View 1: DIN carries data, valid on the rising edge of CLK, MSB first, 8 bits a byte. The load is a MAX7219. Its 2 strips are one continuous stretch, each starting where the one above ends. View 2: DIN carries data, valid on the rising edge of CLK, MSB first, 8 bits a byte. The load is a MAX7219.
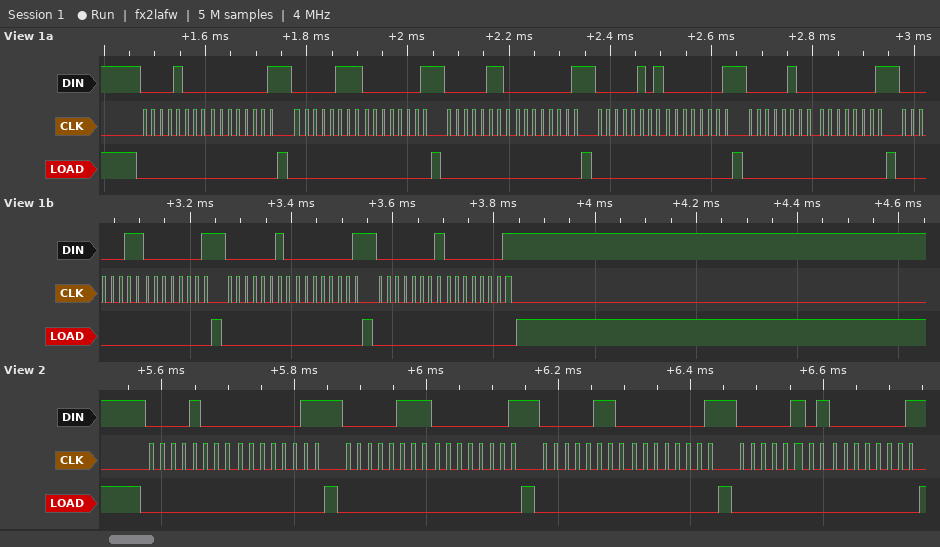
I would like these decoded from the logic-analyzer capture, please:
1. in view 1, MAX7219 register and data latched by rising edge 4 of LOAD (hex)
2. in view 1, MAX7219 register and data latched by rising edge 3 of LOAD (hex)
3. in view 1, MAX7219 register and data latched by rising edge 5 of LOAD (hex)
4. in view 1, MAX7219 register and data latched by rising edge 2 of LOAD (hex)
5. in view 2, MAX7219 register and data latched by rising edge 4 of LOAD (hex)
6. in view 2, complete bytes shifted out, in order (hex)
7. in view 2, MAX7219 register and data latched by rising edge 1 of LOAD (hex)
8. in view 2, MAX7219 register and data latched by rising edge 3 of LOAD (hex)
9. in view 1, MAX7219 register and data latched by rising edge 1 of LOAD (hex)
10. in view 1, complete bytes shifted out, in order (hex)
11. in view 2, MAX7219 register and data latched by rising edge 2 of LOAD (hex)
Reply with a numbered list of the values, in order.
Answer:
1. register 0x5, data 0x01
2. register 0x6, data 0x01
3. register 0x4, data 0x01
4. register 0x7, data 0x01
5. register 0x5, data 0x01
6. 08 03 07 01 06 01 05 01
7. register 0x8, data 0x03
8. register 0x6, data 0x01
9. register 0x8, data 0x01
10. 08 01 07 01 06 01 05 01 04 01 03 01 02 01 01 01
11. register 0x7, data 0x01
